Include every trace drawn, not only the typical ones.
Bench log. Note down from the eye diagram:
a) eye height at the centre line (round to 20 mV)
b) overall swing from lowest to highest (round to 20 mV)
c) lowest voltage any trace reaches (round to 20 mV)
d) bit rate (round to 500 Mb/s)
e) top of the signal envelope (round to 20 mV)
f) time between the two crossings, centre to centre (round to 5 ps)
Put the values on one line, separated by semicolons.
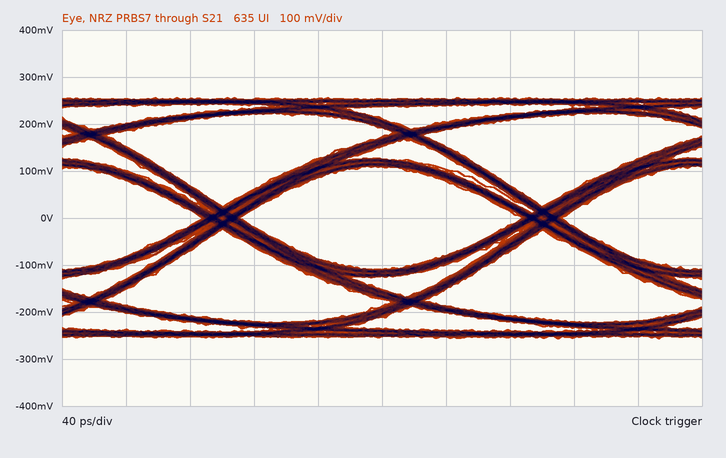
220 mV; 520 mV; -260 mV; 5.0 Gb/s; 260 mV; 200 ps
